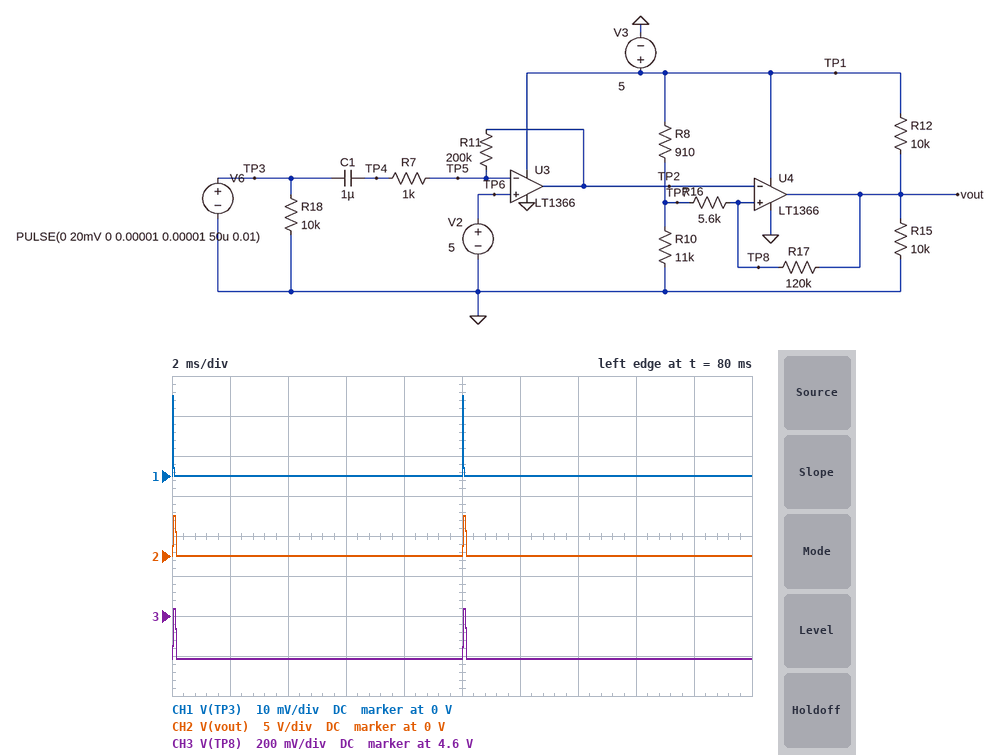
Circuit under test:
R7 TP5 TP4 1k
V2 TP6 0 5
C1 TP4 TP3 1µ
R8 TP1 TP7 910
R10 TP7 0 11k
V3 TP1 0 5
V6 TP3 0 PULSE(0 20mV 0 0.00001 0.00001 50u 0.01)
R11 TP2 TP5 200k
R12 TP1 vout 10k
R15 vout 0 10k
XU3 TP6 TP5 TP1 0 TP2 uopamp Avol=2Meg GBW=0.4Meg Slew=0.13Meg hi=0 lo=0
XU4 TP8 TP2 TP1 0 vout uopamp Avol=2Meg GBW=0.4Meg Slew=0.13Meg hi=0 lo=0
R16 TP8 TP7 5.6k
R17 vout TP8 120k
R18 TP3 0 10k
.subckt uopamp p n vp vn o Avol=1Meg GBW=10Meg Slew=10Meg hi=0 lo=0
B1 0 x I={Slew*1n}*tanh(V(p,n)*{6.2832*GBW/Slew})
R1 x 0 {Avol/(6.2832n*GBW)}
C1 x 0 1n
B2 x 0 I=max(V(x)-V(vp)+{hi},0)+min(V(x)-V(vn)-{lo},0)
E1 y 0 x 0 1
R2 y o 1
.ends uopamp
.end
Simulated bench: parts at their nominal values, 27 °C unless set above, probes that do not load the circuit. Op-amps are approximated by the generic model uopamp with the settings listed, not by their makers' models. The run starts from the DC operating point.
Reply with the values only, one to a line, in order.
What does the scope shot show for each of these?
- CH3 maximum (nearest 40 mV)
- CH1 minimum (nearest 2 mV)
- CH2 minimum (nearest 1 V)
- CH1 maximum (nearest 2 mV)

4.64 V
0 V
0 V
20 mV
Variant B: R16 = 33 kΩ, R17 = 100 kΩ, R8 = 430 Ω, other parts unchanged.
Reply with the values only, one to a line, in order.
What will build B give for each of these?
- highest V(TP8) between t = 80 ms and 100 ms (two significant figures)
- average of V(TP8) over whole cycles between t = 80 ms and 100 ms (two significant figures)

4.9 V
3.6 V
